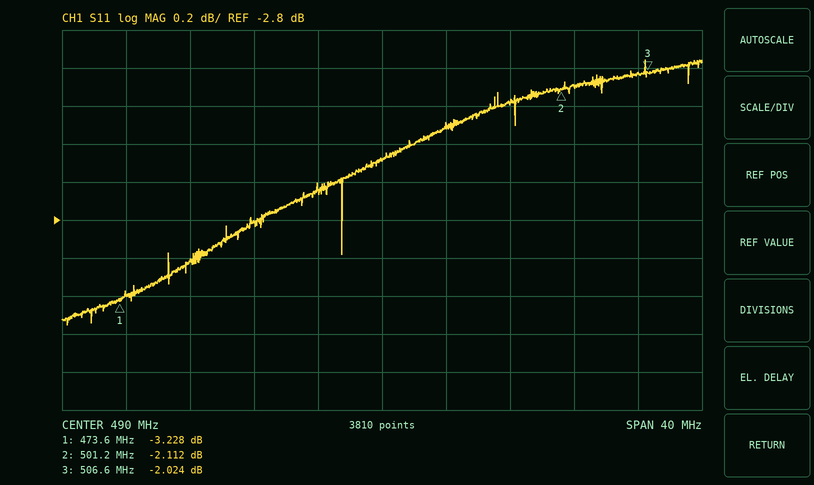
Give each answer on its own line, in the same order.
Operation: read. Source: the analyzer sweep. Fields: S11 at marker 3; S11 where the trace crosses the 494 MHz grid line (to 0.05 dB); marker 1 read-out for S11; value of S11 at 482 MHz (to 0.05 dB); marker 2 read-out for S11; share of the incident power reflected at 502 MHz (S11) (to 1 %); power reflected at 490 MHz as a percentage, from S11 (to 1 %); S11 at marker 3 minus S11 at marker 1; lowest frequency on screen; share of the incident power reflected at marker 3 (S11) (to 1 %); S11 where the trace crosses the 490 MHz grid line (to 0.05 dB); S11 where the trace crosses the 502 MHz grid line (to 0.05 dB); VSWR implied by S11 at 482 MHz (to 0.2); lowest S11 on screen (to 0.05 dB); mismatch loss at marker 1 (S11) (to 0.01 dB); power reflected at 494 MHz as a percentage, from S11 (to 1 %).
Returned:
-2.024 dB
-2.30 dB
-3.228 dB
-2.80 dB
-2.112 dB
62 %
56 %
1.204 dB
470 MHz
63 %
-2.50 dB
-2.10 dB
6.2
-3.35 dB
2.80 dB
59 %
